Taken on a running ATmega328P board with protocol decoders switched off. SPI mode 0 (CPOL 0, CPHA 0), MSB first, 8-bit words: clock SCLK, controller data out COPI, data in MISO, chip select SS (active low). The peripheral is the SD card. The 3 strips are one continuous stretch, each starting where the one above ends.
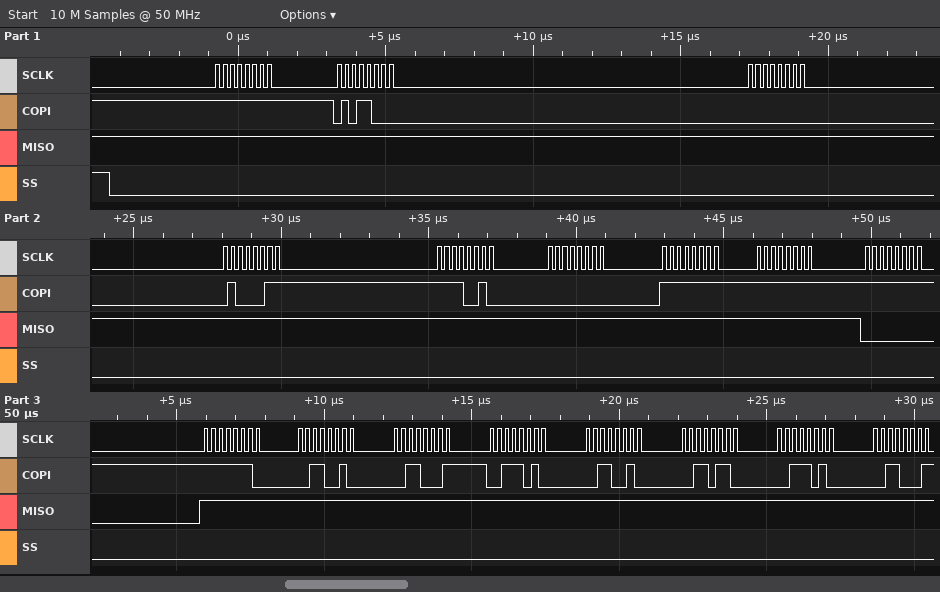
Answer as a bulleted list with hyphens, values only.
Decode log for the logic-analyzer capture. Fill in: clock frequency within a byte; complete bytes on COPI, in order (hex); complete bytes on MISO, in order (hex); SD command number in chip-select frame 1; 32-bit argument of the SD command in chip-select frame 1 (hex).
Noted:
- 4 MHz
- FF 58 00 43 F2 00 FF FF FF FE 32 31 3A 32 36 3A 31
- FF FF FF FF FF FF FF FF 00 FF FF FF FF FF FF FF FF
- CMD24
- 0x0043F200
